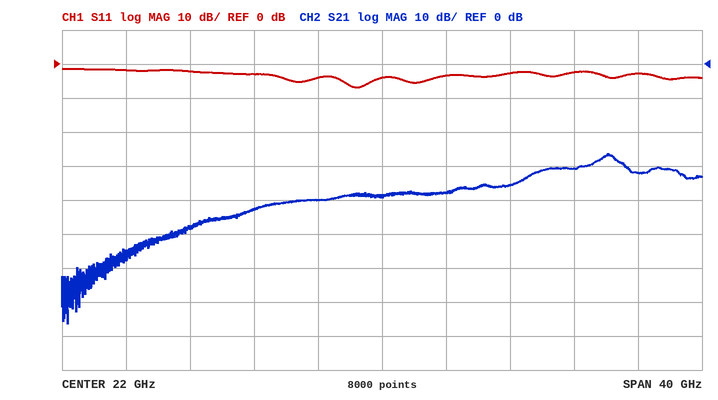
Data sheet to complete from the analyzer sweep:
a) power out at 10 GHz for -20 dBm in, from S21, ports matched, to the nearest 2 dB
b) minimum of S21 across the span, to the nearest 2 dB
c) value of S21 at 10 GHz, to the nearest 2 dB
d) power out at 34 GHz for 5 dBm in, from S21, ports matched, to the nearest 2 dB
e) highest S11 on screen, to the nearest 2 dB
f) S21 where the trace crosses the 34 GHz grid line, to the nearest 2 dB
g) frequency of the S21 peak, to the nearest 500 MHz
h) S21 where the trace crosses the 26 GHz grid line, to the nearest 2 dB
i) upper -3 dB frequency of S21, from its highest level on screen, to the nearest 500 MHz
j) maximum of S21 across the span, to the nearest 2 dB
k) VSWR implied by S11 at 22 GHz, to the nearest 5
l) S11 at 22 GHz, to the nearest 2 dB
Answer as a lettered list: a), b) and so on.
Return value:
a) -68 dBm
b) -76 dB
c) -48 dB
d) -26 dBm
e) -2 dB
f) -30 dB
g) 36.0 GHz
h) -38 dB
i) 37.0 GHz
j) -26 dB
k) 5
l) -4 dB
